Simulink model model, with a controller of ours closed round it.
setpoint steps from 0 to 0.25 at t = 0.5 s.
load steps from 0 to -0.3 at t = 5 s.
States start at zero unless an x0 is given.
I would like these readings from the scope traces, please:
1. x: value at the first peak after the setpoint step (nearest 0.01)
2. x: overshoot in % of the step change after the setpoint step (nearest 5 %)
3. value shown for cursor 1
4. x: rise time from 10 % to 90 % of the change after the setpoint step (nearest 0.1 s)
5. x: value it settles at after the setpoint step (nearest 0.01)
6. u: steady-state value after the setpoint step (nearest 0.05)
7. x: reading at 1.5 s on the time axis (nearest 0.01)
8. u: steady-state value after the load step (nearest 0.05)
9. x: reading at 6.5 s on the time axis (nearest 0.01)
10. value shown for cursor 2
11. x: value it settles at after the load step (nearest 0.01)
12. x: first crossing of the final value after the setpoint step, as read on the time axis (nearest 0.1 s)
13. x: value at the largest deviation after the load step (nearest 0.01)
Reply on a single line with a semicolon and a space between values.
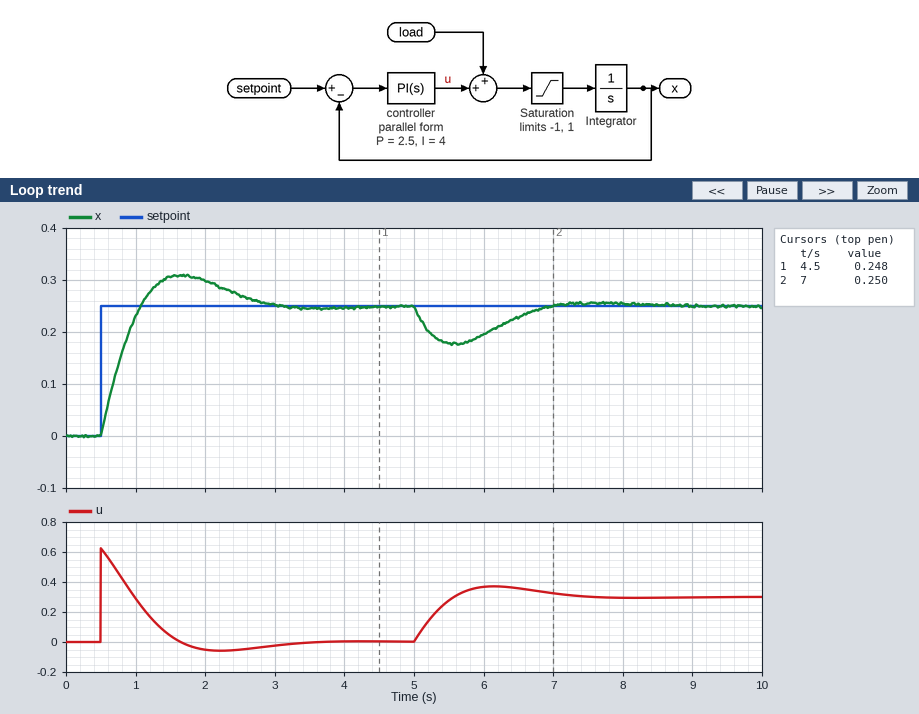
0.31; 25 %; 0.248; 0.4 s; 0.25; 0.00; 0.31; 0.30; 0.23; 0.250; 0.25; 1.1 s; 0.18
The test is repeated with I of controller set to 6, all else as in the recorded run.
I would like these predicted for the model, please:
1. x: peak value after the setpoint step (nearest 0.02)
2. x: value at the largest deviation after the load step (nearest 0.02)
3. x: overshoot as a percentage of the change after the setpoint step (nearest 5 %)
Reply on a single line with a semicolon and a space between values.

0.32; 0.18; 30 %
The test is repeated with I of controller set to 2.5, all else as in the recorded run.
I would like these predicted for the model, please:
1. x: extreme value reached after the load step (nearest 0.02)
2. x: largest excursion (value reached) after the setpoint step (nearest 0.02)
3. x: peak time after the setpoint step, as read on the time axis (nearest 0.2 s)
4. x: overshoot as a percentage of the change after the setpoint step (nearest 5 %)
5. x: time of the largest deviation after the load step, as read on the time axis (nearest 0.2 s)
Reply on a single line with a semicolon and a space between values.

0.16; 0.30; 1.8 s; 20 %; 5.6 s
